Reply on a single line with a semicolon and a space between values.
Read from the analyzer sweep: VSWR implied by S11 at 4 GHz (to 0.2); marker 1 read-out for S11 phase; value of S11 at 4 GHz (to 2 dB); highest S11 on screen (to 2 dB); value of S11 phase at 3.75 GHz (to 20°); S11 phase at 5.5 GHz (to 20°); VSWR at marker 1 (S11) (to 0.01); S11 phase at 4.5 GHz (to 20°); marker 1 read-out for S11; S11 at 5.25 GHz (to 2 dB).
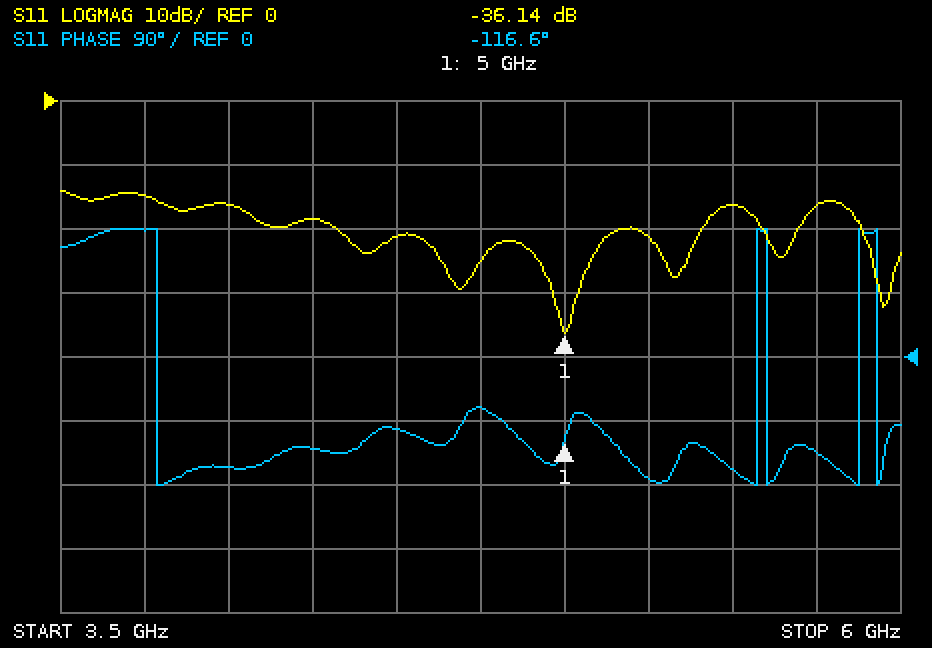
1.4; -116.6°; -16 dB; -14 dB; 180°; -160°; 1.03; -100°; -36.14 dB; -22 dB
